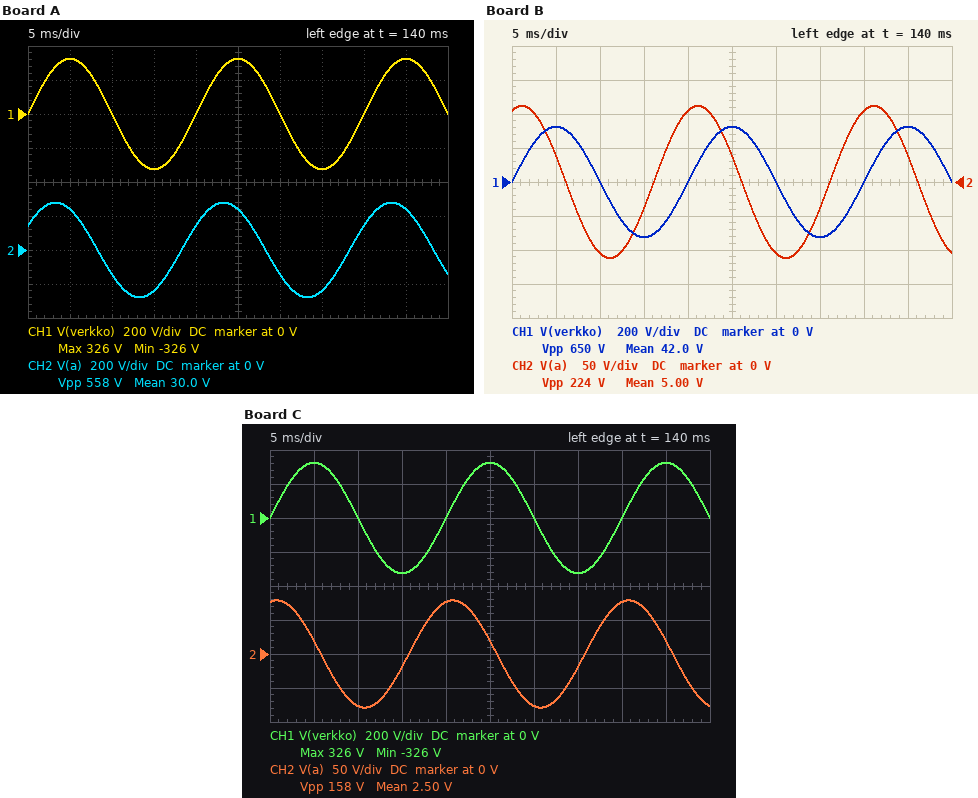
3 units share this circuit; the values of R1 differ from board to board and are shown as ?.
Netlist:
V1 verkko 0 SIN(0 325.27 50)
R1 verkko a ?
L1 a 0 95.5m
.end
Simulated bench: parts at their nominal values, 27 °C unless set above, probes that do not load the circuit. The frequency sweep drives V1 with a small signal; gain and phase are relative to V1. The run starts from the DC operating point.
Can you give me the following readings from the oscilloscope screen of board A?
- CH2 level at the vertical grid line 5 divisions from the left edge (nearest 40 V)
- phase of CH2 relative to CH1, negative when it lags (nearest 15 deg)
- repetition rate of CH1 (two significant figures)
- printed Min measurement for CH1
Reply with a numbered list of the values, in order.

1. 240 V
2. 30 deg
3. 50 Hz
4. -326 V
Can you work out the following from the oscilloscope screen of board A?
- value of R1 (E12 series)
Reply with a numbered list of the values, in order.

1. 18 Ω
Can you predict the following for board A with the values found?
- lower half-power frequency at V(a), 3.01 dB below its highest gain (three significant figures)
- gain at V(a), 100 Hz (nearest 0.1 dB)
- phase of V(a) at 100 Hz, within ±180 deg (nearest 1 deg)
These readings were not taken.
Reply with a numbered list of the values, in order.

1. 30.0 Hz
2. -0.4 dB
3. 17 deg
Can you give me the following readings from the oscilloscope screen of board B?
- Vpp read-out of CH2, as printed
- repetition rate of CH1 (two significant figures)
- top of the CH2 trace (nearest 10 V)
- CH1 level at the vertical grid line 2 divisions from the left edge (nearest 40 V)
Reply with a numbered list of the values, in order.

1. 224 V
2. 50 Hz
3. 110 V
4. 0 V
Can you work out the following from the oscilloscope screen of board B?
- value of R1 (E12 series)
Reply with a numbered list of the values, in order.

1. 82 Ω
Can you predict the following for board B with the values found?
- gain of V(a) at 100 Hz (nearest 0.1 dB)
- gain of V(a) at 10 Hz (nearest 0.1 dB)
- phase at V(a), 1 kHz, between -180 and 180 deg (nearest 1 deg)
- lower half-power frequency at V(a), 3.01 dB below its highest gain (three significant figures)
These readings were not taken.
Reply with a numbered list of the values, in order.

1. -4.6 dB
2. -22.7 dB
3. 8 deg
4. 137 Hz
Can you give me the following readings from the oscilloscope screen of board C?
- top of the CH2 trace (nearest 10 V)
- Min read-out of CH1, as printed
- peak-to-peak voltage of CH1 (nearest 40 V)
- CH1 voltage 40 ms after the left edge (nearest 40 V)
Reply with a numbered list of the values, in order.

1. 80 V
2. -326 V
3. 640 V
4. 0 V
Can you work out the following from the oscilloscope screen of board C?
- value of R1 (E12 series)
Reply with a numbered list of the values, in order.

1. 120 Ω
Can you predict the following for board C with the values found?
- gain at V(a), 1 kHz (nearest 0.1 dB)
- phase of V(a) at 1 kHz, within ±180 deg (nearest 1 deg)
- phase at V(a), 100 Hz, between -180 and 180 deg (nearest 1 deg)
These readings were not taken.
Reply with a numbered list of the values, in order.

1. -0.2 dB
2. 11 deg
3. 63 deg
